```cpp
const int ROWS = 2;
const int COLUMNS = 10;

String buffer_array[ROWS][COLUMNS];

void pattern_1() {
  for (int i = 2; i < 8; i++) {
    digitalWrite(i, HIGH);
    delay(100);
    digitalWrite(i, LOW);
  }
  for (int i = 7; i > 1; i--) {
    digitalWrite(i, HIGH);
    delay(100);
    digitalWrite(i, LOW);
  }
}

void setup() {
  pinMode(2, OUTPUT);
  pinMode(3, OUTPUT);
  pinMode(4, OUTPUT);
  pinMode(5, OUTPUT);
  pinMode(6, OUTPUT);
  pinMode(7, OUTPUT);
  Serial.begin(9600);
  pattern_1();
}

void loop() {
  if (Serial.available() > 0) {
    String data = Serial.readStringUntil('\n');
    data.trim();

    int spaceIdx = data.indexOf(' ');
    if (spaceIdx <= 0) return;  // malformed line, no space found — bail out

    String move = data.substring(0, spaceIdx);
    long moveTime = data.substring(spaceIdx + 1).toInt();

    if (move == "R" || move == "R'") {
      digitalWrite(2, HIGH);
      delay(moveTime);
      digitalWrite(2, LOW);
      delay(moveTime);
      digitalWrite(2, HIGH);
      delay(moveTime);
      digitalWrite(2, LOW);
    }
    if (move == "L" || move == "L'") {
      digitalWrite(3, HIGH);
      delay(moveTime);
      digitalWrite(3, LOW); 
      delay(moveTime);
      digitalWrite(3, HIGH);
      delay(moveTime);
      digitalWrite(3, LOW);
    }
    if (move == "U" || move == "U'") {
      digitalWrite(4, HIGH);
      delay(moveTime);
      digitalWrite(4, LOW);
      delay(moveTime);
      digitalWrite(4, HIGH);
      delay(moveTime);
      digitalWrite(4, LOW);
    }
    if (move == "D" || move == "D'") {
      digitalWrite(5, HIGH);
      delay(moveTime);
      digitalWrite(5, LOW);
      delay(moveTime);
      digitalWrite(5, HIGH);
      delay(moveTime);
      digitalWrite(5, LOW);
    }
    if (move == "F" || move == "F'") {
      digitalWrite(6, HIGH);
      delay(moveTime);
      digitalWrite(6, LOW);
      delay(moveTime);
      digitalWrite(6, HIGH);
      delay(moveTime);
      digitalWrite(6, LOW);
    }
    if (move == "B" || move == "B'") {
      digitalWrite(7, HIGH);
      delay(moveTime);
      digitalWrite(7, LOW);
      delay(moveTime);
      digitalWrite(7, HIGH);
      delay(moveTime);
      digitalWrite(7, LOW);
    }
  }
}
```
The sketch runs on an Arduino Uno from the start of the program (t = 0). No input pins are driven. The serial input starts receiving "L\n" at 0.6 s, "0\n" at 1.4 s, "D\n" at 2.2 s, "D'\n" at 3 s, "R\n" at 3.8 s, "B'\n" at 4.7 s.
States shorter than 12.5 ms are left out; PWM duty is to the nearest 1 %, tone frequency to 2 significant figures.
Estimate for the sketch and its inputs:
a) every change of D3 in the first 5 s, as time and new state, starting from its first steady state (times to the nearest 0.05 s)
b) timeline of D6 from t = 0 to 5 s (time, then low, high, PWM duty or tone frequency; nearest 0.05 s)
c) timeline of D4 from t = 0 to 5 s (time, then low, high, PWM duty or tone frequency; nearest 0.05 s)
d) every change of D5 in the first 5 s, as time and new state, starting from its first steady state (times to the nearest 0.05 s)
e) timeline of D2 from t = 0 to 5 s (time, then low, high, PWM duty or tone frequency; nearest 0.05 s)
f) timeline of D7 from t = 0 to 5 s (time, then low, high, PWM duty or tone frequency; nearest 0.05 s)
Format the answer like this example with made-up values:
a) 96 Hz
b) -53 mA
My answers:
a) 0 s low; 0.1 s high; 0.2 s low; 1 s high; 1.1 s low
b) 0 s low; 0.4 s high; 0.5 s low; 0.7 s high; 0.8 s low
c) 0 s low; 0.2 s high; 0.3 s low; 0.9 s high; 1 s low
d) 0 s low; 0.3 s high; 0.4 s low; 0.8 s high; 0.9 s low
e) 0 s high; 0.1 s low; 1.1 s high; 1.2 s low
f) 0 s low; 0.5 s high; 0.7 s low
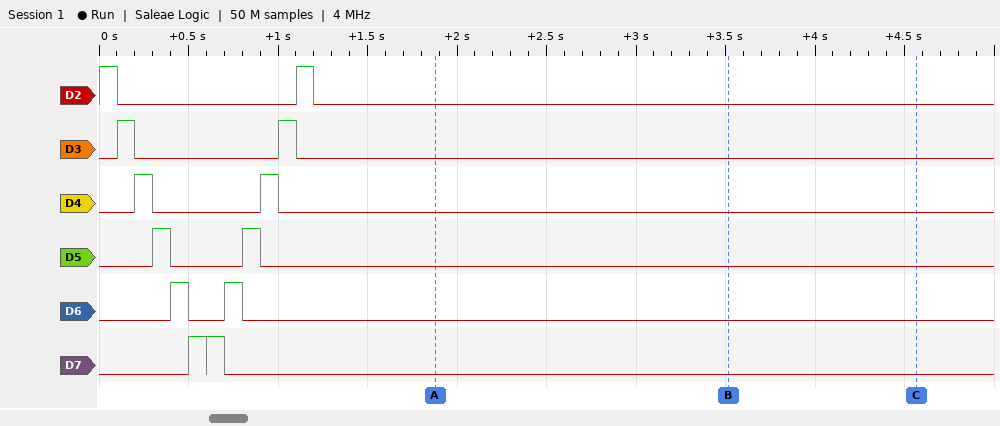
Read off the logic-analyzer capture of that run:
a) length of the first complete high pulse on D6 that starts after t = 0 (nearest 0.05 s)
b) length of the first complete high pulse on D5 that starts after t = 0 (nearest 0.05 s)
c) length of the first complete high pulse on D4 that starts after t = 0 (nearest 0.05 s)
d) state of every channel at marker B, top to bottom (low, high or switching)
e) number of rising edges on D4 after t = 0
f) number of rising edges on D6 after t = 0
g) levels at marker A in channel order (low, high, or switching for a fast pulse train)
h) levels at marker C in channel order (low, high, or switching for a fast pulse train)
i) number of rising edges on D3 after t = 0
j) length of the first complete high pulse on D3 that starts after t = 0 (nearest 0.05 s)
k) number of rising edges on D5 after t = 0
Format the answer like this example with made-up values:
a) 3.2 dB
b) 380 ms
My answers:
a) 0.10 s
b) 0.10 s
c) 0.10 s
d) D2 low, D3 low, D4 low, D5 low, D6 low, D7 low
e) 2
f) 2
g) D2 low, D3 low, D4 low, D5 low, D6 low, D7 low
h) D2 low, D3 low, D4 low, D5 low, D6 low, D7 low
i) 2
j) 0.10 s
k) 2
